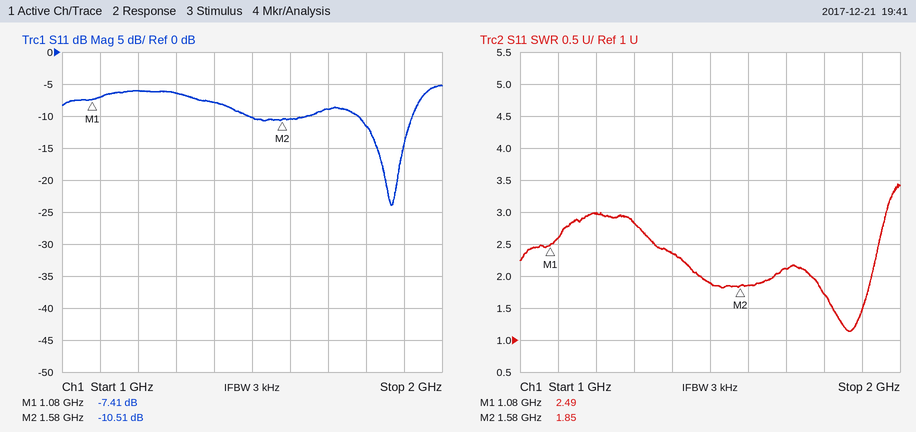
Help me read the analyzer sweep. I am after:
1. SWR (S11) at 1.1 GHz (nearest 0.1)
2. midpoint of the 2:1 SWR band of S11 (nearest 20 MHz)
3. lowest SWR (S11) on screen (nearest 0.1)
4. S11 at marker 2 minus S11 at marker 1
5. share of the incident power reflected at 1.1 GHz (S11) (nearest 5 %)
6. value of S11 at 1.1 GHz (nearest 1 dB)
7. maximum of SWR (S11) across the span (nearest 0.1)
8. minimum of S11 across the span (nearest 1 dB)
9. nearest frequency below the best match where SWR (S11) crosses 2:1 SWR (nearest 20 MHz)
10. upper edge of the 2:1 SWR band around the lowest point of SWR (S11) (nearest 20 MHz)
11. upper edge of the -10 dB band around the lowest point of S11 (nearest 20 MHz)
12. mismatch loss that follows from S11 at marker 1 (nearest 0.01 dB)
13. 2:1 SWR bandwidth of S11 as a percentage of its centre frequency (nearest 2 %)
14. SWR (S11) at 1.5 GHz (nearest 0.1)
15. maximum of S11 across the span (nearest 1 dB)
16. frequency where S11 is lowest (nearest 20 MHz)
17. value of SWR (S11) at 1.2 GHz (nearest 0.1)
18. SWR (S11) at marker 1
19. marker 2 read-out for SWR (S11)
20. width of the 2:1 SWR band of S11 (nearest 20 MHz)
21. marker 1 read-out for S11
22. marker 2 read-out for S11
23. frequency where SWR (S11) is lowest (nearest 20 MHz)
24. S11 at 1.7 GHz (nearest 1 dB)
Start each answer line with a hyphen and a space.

- 2.6
- 1.84 GHz
- 1.1
- -3.10 dB
- 20 %
- -7 dB
- 3.4
- -24 dB
- 1.76 GHz
- 1.92 GHz
- 1.92 GHz
- 0.87 dB
- 8 %
- 1.9
- -5 dB
- 1.86 GHz
- 3.0
- 2.49
- 1.85
- 160 MHz
- -7.41 dB
- -10.51 dB
- 1.86 GHz
- -9 dB
